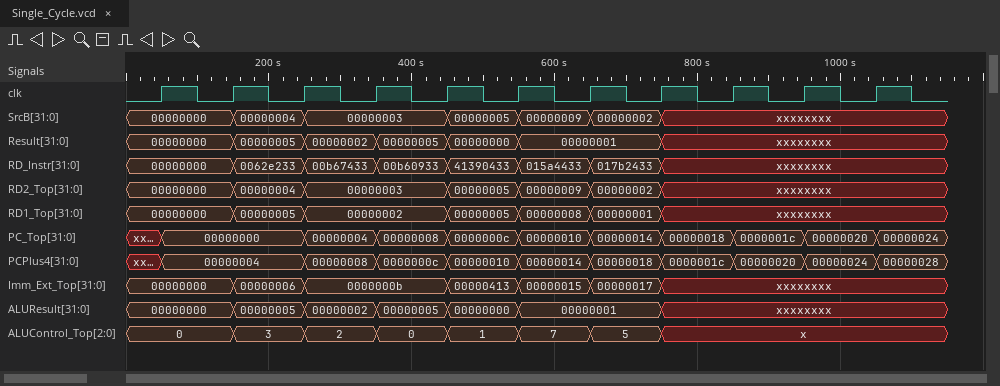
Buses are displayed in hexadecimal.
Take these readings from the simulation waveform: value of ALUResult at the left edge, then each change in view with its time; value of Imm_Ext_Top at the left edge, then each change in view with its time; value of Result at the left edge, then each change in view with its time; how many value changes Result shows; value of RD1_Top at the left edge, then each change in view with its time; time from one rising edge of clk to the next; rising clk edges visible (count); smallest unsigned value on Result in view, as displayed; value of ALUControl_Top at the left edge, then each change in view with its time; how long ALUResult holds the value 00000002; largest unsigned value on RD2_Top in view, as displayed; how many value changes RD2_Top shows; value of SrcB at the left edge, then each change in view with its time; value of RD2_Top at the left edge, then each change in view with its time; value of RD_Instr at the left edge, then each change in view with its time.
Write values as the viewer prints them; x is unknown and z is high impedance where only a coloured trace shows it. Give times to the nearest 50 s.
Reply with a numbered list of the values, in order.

1. 00000000, 00000005 at 150 s, 00000002 at 250 s, 00000005 at 350 s, 00000000 at 450 s, 00000001 at 550 s, xxxxxxxx at 750 s
2. 00000000, 00000006 at 150 s, 0000000b at 250 s, 00000413 at 450 s, 00000015 at 550 s, 00000017 at 650 s, xxxxxxxx at 750 s
3. 00000000, 00000005 at 150 s, 00000002 at 250 s, 00000005 at 350 s, 00000000 at 450 s, 00000001 at 550 s, xxxxxxxx at 750 s
4. 6
5. 00000000, 00000005 at 150 s, 00000002 at 250 s, 00000005 at 450 s, 00000008 at 550 s, 00000001 at 650 s, xxxxxxxx at 750 s
6. 100 s
7. 11
8. 00000000
9. 0, 3 at 150 s, 2 at 250 s, 0 at 350 s, 1 at 450 s, 7 at 550 s, 5 at 650 s, x at 750 s
10. 100 s
11. 00000009
12. 6
13. 00000000, 00000004 at 150 s, 00000003 at 250 s, 00000005 at 450 s, 00000009 at 550 s, 00000002 at 650 s, xxxxxxxx at 750 s
14. 00000000, 00000004 at 150 s, 00000003 at 250 s, 00000005 at 450 s, 00000009 at 550 s, 00000002 at 650 s, xxxxxxxx at 750 s
15. 00000000, 0062e233 at 150 s, 00b67433 at 250 s, 00b60933 at 350 s, 41390433 at 450 s, 015a4433 at 550 s, 017b2433 at 650 s, xxxxxxxx at 750 s
